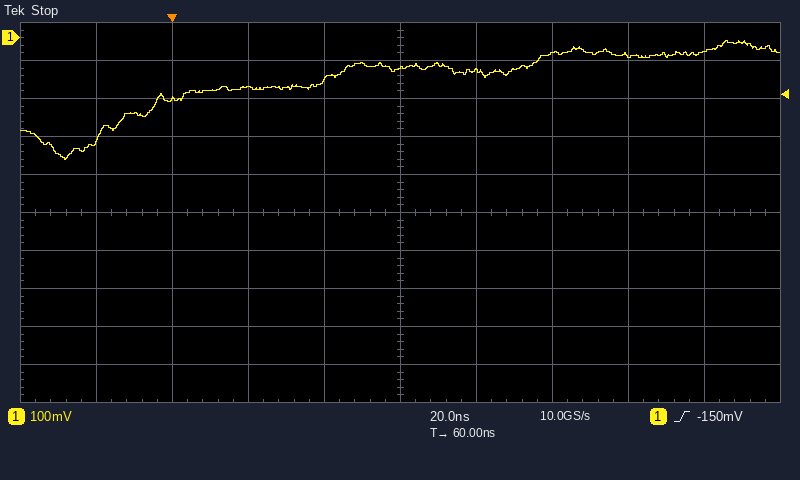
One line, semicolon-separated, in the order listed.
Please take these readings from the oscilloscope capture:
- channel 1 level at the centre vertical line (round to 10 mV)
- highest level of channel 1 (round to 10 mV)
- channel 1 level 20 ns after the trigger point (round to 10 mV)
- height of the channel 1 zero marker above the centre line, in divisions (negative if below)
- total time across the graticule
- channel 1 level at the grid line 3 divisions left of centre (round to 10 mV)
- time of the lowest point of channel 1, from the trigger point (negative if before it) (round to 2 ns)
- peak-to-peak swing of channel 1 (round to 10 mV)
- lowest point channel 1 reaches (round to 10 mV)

-80 mV; -10 mV; -130 mV; +4.6 div; 200 ns; -160 mV; -28 ns; 310 mV; -320 mV
